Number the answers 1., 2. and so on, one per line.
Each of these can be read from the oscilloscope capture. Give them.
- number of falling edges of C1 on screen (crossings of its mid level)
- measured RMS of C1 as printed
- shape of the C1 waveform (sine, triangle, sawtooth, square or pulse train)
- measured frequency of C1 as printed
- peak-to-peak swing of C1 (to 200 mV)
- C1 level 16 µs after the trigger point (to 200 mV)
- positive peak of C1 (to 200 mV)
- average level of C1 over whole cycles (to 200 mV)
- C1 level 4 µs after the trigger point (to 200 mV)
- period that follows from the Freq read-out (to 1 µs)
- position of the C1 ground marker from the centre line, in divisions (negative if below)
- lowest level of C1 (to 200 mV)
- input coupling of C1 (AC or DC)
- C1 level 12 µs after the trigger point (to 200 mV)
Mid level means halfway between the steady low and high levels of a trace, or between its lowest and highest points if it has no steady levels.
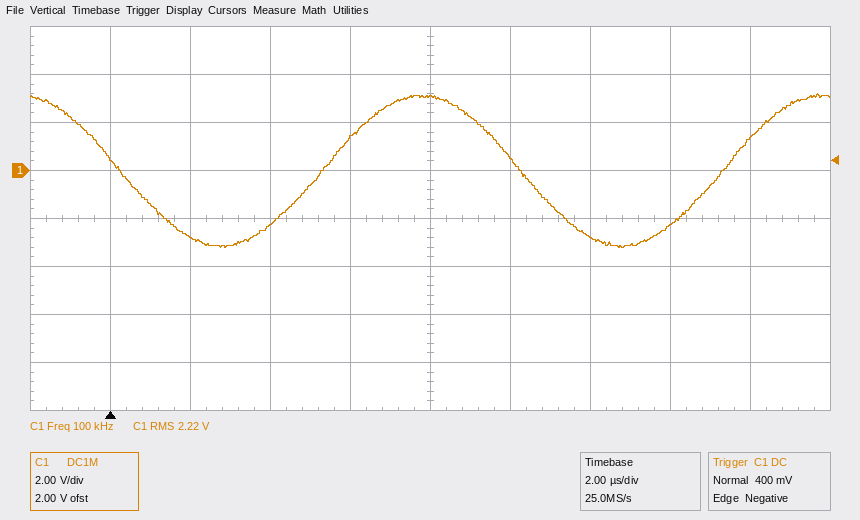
1. 2
2. 2.22 V
3. sine
4. 100 kHz
5. 6.4 V
6. 1.4 V
7. 3.2 V
8. 0.0 V
9. -2.2 V
10. 10 µs
11. +1.0 div
12. -3.2 V
13. DC
14. -2.8 V
